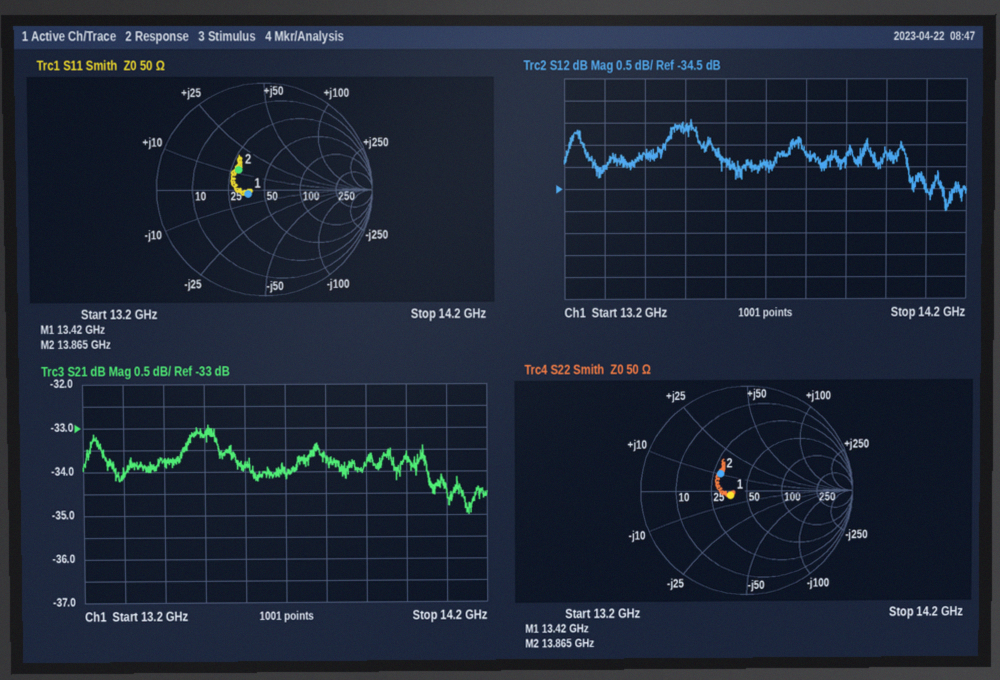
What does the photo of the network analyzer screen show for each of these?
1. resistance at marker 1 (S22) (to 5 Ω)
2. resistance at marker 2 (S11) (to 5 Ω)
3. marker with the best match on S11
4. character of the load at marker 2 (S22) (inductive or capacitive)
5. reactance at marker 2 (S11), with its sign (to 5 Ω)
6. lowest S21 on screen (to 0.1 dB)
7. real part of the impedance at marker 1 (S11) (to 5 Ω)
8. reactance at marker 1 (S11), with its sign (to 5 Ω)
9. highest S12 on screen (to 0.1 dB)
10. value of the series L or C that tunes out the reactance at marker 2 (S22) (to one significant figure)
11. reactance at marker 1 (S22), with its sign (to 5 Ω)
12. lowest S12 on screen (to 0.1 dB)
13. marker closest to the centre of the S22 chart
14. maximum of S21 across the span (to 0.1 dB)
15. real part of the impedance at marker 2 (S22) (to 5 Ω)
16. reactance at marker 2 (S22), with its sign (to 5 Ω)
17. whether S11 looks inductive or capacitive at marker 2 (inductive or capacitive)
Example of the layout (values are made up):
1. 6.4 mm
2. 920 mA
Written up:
1. 35 Ω
2. 30 Ω
3. marker 1
4. inductive
5. +10 Ω
6. -35.0 dB
7. 35 Ω
8. -5 Ω
9. -32.9 dB
10. 1 pF
11. -5 Ω
12. -35.0 dB
13. marker 1
14. -32.9 dB
15. 30 Ω
16. +10 Ω
17. inductive
